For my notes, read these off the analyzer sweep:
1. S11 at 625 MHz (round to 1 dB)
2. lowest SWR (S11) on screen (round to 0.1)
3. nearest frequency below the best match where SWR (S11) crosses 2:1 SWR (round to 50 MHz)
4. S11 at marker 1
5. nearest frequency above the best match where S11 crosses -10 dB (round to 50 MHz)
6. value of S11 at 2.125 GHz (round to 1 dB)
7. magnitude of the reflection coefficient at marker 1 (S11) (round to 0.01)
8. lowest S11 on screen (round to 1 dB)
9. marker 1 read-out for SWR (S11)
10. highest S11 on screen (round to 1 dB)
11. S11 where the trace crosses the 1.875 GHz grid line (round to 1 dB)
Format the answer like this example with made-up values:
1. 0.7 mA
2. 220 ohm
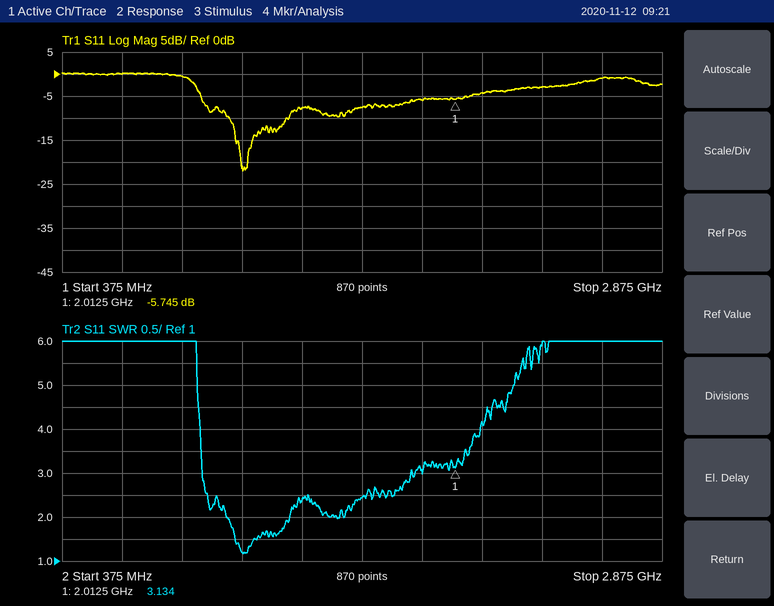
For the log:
1. 0 dB
2. 1.2
3. 1.05 GHz
4. -5.745 dB
5. 1.30 GHz
6. -4 dB
7. 0.52
8. -22 dB
9. 3.134
10. 0 dB
11. -6 dB
